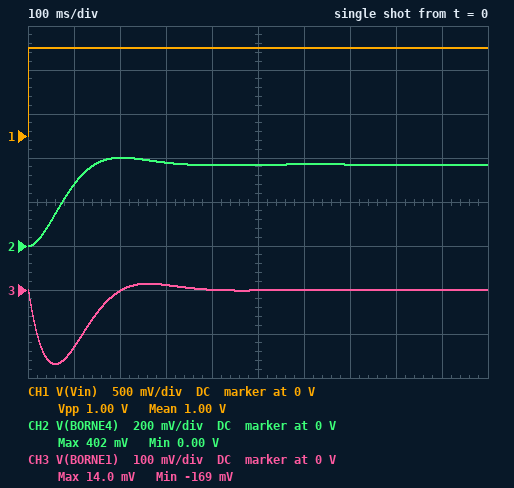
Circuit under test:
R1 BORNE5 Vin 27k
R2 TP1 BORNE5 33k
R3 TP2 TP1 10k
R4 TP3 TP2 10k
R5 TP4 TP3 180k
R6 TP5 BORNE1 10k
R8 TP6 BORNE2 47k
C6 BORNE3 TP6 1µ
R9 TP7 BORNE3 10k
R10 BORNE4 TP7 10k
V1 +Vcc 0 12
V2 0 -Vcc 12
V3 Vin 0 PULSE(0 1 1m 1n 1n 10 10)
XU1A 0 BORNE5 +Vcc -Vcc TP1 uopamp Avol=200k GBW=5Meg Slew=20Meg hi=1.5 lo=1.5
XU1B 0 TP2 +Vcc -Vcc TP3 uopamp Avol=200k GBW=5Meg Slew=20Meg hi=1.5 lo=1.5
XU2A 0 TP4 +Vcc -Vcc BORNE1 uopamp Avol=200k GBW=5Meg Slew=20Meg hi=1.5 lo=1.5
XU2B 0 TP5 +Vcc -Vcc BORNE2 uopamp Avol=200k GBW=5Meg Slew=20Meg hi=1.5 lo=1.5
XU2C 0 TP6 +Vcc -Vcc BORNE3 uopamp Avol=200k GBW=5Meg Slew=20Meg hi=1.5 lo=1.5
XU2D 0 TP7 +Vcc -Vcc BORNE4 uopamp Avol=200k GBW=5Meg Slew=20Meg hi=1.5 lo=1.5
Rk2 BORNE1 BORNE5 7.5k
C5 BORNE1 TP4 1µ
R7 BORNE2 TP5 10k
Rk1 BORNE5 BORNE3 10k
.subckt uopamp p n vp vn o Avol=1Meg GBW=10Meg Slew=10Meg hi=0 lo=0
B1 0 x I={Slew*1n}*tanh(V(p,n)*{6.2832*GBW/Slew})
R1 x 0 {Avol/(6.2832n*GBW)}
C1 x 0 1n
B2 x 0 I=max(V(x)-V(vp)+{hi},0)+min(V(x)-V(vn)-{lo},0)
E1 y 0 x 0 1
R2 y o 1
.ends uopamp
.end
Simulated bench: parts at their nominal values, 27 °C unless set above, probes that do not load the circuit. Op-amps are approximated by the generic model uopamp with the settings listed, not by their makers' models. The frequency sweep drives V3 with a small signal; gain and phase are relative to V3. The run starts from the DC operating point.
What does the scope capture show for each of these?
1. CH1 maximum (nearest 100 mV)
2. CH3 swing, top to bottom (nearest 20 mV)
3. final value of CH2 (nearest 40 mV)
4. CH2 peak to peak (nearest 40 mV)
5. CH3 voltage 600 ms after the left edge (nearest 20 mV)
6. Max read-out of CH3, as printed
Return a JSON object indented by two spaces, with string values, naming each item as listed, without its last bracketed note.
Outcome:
{
  "CH1 maximum": "1.0 V",
  "CH3 swing, top to bottom": "180 mV",
  "final value of CH2": "360 mV",
  "CH2 peak to peak": "400 mV",
  "CH3 voltage 600 ms after the left edge": "0 V",
  "Max read-out of CH3, as printed": "14.0 mV"
}
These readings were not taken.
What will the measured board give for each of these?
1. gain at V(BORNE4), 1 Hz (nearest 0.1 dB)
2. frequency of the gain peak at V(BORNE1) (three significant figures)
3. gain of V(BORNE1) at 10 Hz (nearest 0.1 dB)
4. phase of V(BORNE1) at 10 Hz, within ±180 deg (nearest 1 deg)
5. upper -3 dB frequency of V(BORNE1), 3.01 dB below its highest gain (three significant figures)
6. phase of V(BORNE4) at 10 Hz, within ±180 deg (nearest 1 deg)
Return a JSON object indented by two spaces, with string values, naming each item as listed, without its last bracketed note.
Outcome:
{
  "gain at V(BORNE4), 1 Hz": "-8.5 dB",
  "frequency of the gain peak at V(BORNE1)": "3.14 Hz",
  "gain of V(BORNE1) at 10 Hz": "-19.2 dB",
  "phase of V(BORNE1) at 10 Hz, within ±180 deg": "113 deg",
  "upper -3 dB frequency of V(BORNE1), 3.01 dB below its highest gain": "5.64 Hz",
  "phase of V(BORNE4) at 10 Hz, within ±180 deg": "-157 deg"
}
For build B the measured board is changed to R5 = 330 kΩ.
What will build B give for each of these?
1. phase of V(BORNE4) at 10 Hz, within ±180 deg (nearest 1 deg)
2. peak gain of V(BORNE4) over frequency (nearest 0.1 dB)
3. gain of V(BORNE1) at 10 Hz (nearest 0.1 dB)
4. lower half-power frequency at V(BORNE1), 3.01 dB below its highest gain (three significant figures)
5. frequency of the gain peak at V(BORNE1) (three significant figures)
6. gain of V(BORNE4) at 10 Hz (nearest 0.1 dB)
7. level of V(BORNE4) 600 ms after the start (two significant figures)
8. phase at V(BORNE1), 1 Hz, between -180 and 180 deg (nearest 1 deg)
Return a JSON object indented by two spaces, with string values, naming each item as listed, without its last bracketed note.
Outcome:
{
  "phase of V(BORNE4) at 10 Hz, within ±180 deg": "-167 deg",
  "peak gain of V(BORNE4) over frequency": "-6.8 dB",
  "gain of V(BORNE1) at 10 Hz": "-24.3 dB",
  "lower half-power frequency at V(BORNE1), 3.01 dB below its highest gain": "1.49 Hz",
  "frequency of the gain peak at V(BORNE1)": "2.32 Hz",
  "gain of V(BORNE4) at 10 Hz": "-33.7 dB",
  "level of V(BORNE4) 600 ms after the start": "370 mV",
  "phase at V(BORNE1), 1 Hz, between -180 and 180 deg": "-116 deg"
}
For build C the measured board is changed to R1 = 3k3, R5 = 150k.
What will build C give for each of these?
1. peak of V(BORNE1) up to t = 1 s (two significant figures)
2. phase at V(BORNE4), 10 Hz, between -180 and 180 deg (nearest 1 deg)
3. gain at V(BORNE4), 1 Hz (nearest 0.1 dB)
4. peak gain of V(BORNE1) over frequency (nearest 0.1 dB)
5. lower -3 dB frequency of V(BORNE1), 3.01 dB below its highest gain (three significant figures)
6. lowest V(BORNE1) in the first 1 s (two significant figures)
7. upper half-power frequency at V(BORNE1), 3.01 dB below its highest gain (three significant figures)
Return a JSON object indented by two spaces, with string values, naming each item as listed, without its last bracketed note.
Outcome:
{
  "peak of V(BORNE1) up to t = 1 s": "79 mV",
  "phase at V(BORNE4), 10 Hz, between -180 and 180 deg": "-152 deg",
  "gain at V(BORNE4), 1 Hz": "9.7 dB",
  "peak gain of V(BORNE1) over frequency": "7.1 dB",
  "lower -3 dB frequency of V(BORNE1), 3.01 dB below its highest gain": "1.83 Hz",
  "lowest V(BORNE1) in the first 1 s": "-1.4 V",
  "upper half-power frequency at V(BORNE1), 3.01 dB below its highest gain": "6.49 Hz"
}
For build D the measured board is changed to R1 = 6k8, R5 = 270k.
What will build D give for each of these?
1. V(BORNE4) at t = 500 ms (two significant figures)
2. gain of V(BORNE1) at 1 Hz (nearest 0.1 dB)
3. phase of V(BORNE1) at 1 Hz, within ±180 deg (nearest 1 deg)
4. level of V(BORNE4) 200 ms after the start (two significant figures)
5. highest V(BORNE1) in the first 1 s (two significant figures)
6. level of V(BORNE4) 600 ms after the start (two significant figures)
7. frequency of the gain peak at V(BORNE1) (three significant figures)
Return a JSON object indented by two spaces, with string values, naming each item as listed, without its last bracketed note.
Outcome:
{
  "V(BORNE4) at t = 500 ms": "1.4 V",
  "gain of V(BORNE1) at 1 Hz": "-6.7 dB",
  "phase of V(BORNE1) at 1 Hz, within ±180 deg": "-115 deg",
  "level of V(BORNE4) 200 ms after the start": "1.7 V",
  "highest V(BORNE1) in the first 1 s": "96 mV",
  "level of V(BORNE4) 600 ms after the start": "1.5 V",
  "frequency of the gain peak at V(BORNE1)": "2.57 Hz"
}
